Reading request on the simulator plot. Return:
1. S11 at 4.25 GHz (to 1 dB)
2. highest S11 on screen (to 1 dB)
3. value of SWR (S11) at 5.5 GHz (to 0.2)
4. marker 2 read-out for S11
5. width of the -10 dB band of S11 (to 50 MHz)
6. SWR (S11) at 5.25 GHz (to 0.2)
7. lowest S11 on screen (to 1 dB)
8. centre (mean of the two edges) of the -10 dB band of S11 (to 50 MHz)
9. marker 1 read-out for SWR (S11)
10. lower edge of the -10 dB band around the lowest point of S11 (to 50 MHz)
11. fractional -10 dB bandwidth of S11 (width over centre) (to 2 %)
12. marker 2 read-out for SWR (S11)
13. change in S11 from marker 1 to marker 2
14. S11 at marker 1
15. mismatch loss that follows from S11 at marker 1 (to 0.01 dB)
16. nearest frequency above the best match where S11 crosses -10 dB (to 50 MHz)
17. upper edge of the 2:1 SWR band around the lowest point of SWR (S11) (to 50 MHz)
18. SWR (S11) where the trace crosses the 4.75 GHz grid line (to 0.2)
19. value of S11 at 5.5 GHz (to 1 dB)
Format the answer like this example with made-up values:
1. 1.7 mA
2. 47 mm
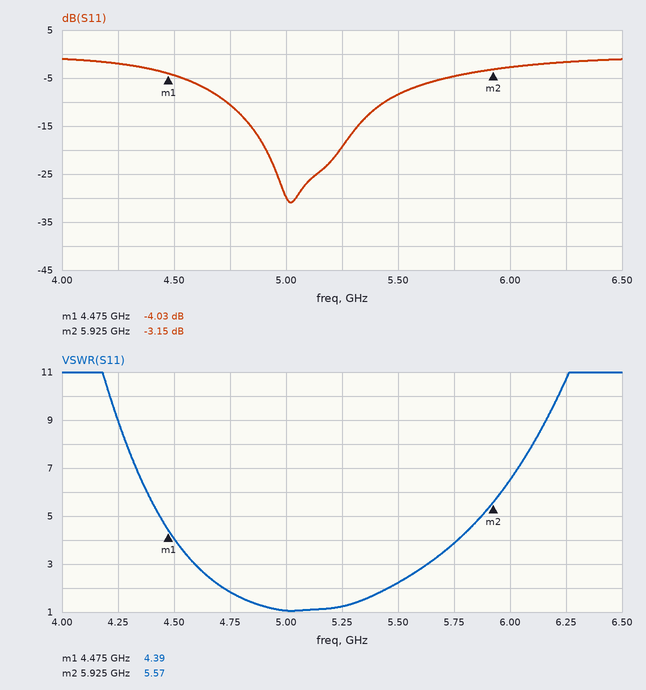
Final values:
1. -2 dB
2. -1 dB
3. 2.2
4. -3.15 dB
5. 700 MHz
6. 1.2
7. -31 dB
8. 5.10 GHz
9. 4.39
10. 4.75 GHz
11. 14 %
12. 5.57
13. 0.88 dB
14. -4.03 dB
15. 2.19 dB
16. 5.45 GHz
17. 5.45 GHz
18. 1.8
19. -8 dB
